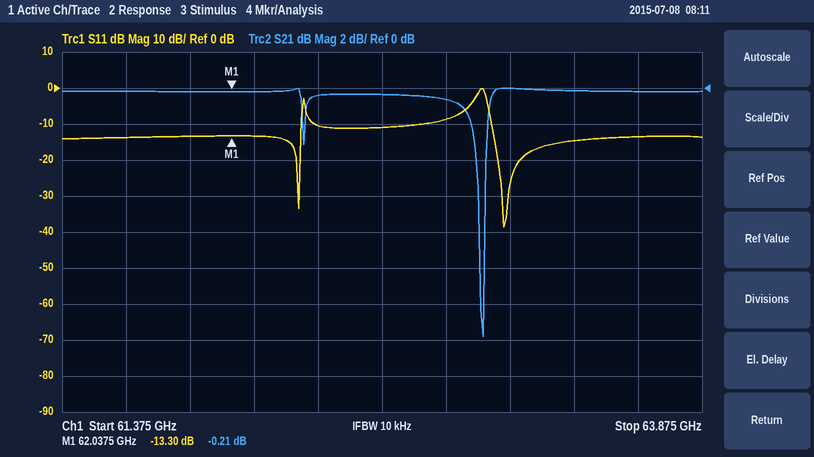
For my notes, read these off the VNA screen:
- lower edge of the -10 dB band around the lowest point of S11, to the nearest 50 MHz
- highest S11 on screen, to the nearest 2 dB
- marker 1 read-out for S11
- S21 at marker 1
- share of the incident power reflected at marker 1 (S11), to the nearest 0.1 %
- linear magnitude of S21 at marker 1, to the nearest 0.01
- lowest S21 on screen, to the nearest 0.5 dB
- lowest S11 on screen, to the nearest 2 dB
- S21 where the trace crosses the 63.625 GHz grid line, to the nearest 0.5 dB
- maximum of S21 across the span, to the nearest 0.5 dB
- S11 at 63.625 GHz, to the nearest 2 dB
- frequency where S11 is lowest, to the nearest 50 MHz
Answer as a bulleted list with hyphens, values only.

- 63.05 GHz
- 0 dB
- -13.30 dB
- -0.21 dB
- 4.7 %
- 0.98
- -14.0 dB
- -38 dB
- 0.0 dB
- 0.0 dB
- -14 dB
- 63.10 GHz
